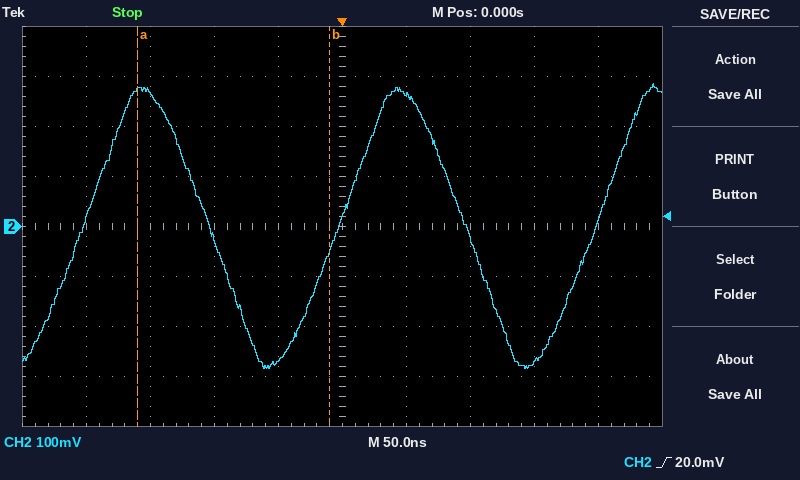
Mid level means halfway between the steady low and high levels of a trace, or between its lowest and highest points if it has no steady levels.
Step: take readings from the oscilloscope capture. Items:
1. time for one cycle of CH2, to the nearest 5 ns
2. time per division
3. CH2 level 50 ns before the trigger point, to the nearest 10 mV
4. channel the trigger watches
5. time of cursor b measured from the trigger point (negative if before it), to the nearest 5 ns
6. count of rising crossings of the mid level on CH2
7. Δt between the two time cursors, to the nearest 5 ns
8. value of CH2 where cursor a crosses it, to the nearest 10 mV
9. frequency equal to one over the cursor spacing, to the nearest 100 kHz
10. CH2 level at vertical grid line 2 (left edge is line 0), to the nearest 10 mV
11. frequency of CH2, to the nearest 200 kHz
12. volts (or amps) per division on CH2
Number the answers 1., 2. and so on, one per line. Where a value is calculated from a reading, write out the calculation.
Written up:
1. 200 ns
2. 50 ns
3. -270 mV
4. CH2
5. -10 ns
6. 3
7. 150 ns
8. 270 mV
9. 1 / 150 ns ≈ 6.7 MHz
10. 270 mV
11. 1 / 200 ns ≈ 5.0 MHz
12. 100 mV
